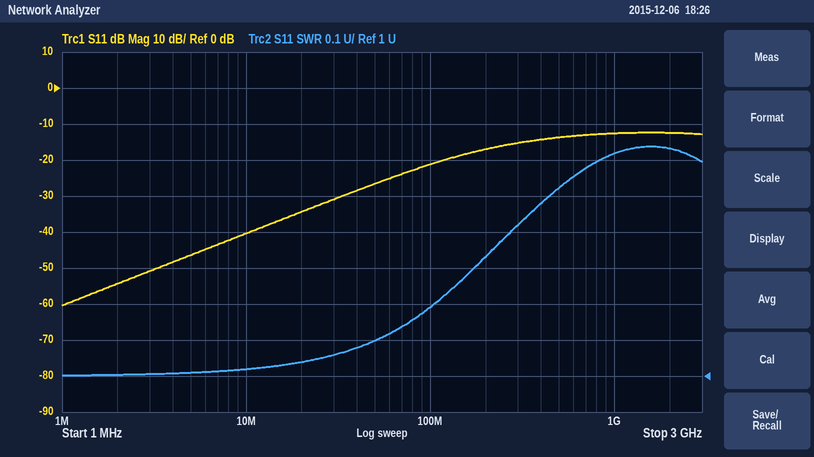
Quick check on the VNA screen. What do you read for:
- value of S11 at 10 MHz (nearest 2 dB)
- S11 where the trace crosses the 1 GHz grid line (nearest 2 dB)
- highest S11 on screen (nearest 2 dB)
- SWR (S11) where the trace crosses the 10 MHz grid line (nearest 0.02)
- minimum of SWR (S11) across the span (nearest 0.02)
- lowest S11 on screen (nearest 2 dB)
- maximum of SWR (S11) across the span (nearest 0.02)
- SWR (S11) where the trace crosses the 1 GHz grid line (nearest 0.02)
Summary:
-40 dB
-12 dB
-12 dB
1.02
1.00
-60 dB
1.64
1.62
